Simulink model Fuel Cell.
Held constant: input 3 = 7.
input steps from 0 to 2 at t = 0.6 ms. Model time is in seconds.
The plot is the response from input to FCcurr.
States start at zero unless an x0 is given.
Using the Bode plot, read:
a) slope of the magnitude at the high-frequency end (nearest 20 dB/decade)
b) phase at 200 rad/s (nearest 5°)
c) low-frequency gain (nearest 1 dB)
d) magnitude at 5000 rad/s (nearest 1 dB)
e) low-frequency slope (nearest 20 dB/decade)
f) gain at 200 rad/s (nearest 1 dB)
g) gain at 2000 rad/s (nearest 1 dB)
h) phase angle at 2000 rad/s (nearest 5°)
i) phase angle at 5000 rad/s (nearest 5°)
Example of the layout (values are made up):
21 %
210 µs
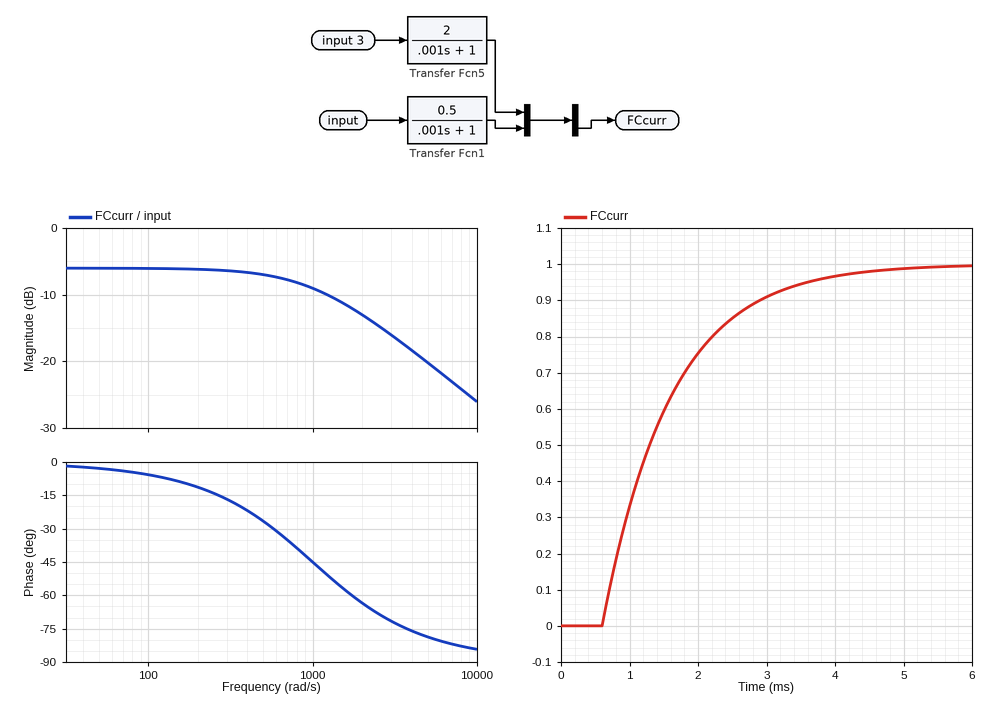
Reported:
-20 dB/decade
-10°
-6 dB
-20 dB
0 dB/decade
-6 dB
-13 dB
-65°
-80°
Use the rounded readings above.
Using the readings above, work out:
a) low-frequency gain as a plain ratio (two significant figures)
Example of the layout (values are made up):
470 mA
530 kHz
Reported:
0.50
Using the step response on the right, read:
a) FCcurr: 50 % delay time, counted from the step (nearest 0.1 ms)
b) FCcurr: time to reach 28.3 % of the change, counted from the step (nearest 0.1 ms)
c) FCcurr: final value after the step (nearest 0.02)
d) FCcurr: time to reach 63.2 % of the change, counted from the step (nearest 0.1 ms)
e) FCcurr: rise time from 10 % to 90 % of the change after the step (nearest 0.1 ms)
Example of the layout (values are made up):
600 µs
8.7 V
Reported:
0.7 ms
0.3 ms
1.00
1.0 ms
2.2 ms
